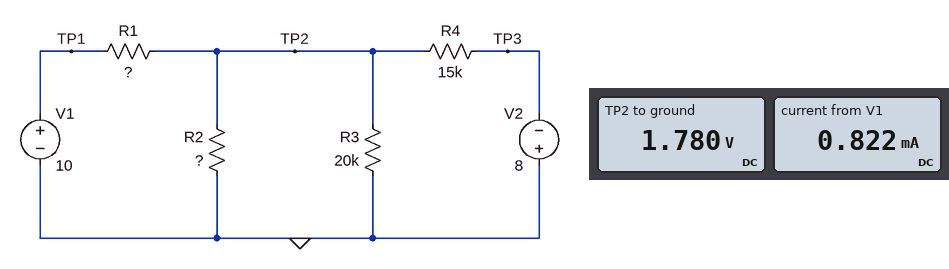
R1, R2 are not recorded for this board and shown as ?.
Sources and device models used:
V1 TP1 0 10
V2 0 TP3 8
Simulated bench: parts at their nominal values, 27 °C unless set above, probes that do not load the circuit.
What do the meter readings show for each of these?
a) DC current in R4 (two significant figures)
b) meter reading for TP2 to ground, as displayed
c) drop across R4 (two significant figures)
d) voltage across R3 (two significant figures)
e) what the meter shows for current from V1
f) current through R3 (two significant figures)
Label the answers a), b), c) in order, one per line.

a) 650 µA
b) 1.780 V
c) 9.8 V
d) 1.8 V
e) 0.822 mA
f) 89 µA
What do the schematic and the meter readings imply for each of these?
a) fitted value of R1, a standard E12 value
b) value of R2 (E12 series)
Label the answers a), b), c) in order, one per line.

a) 10 kΩ
b) 22 kΩ
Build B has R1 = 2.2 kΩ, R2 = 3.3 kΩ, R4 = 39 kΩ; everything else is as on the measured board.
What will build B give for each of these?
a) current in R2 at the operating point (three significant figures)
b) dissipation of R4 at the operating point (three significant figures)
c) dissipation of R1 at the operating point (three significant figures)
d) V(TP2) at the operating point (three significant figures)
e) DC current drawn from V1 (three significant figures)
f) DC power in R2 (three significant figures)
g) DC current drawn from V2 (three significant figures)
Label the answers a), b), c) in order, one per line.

a) 1.58 mA
b) 4.47 mW
c) 10.4 mW
d) 5.21 V
e) 2.18 mA
f) 8.22 mW
g) 339 µA
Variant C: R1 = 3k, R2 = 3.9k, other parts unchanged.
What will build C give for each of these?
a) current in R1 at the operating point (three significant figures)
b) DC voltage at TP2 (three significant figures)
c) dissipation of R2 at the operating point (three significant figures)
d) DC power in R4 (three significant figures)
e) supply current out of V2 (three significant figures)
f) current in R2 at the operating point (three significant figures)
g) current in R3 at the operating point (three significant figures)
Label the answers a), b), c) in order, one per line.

a) 2.01 mA
b) 3.96 V
c) 4.03 mW
d) 9.54 mW
e) 798 µA
f) 1.02 mA
g) 198 µA
